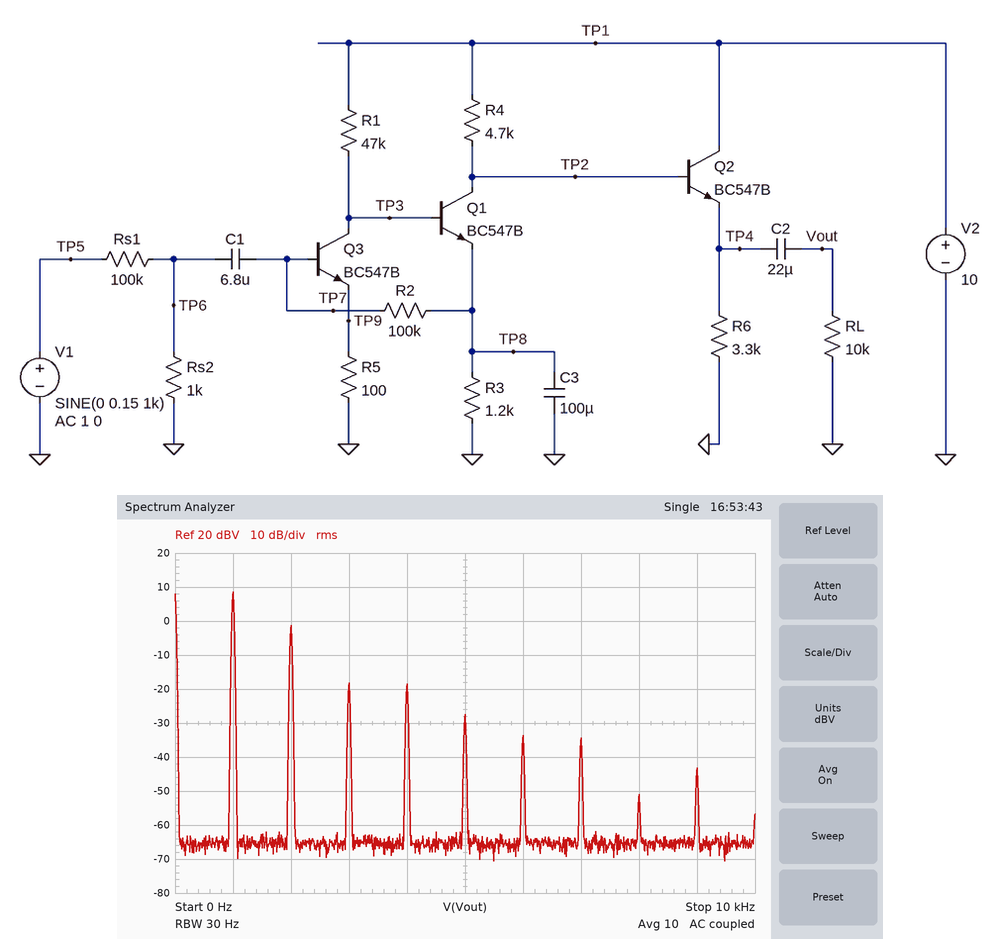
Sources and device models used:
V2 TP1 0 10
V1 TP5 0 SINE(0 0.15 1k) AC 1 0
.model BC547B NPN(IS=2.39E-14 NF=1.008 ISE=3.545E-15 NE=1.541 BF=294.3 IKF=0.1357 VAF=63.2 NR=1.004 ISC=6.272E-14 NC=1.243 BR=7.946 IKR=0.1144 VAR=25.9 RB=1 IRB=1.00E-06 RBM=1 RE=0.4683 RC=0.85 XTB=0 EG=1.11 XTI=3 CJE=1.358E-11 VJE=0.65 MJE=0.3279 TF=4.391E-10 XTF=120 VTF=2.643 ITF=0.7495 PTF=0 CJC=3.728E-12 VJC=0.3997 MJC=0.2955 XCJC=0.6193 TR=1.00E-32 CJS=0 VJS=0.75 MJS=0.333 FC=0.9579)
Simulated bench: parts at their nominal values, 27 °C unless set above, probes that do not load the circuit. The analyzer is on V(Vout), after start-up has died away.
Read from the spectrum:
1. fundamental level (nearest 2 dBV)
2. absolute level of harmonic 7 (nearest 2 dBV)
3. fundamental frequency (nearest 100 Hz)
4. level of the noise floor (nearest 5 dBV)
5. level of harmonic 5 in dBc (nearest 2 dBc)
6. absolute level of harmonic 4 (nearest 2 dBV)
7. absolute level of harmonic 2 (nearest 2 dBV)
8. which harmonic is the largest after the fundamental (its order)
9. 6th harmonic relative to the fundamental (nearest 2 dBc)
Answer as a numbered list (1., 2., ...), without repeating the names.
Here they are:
1. 8 dBV
2. -34 dBV
3. 1.0 kHz
4. -65 dBV
5. -36 dBc
6. -18 dBV
7. -2 dBV
8. 2
9. -42 dBc
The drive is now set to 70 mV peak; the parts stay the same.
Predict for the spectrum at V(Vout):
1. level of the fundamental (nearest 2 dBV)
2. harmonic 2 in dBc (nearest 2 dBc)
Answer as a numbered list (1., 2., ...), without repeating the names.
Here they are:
1. 6 dBV
2. -22 dBc
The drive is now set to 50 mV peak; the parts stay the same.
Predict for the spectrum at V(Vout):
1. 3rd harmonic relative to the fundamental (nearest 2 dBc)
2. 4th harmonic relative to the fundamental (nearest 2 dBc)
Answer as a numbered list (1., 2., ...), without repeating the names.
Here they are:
1. -38 dBc
2. -54 dBc
